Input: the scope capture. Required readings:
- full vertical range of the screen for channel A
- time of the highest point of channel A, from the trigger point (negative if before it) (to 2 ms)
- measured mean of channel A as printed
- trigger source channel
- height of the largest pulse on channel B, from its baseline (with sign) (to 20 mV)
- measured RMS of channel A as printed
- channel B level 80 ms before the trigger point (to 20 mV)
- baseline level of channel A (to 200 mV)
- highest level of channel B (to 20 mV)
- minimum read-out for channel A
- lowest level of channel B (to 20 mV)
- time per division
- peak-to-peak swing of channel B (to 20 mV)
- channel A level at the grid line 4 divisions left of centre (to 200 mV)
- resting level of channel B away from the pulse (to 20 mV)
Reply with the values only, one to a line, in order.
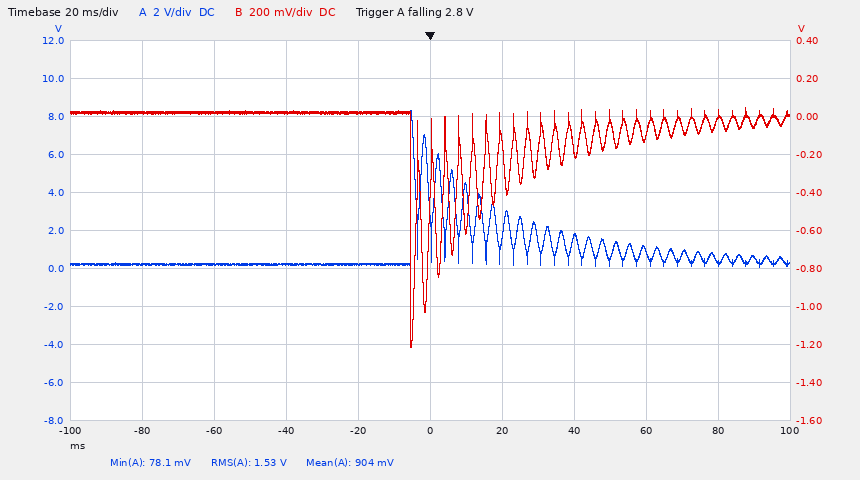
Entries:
20 V
-6 ms
904 mV
channel A
-1.24 V
1.53 V
20 mV
200 mV
40 mV
78.1 mV
-1.22 V
20 ms
1.26 V
200 mV
20 mV
